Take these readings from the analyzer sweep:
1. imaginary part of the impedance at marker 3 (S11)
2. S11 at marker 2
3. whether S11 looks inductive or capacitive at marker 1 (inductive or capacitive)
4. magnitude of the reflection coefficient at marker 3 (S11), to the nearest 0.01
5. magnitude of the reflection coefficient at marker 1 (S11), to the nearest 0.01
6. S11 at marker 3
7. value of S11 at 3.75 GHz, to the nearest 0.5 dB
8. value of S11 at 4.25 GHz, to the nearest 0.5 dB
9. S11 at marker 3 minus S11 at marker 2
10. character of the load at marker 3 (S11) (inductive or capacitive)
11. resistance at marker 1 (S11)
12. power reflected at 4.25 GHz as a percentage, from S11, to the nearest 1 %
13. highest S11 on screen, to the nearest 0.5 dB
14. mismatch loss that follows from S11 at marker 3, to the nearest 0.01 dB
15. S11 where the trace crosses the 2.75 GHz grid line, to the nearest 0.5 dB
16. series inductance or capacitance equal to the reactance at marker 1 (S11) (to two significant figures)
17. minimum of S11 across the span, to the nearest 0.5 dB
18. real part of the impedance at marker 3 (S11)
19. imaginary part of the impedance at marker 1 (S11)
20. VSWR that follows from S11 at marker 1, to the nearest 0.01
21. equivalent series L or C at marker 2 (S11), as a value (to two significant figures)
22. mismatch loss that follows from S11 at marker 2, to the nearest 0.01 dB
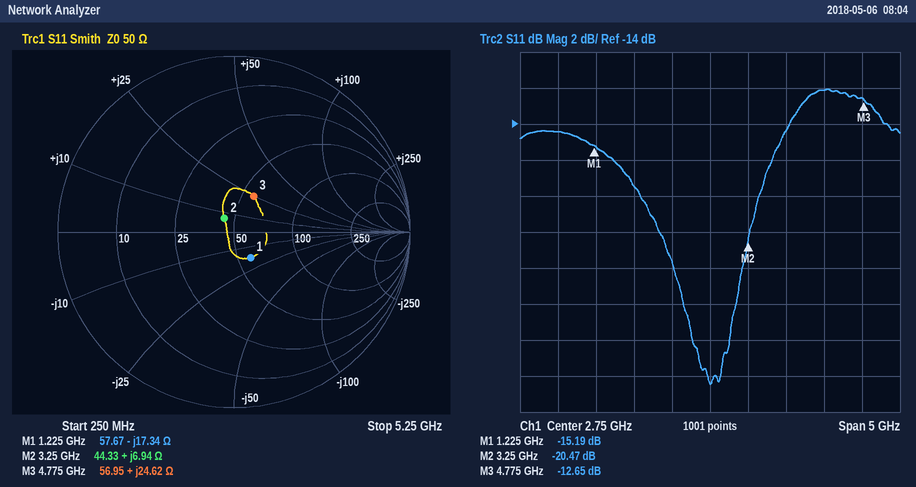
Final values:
+24.62 Ω
-20.47 dB
capacitive
0.23
0.17
-12.65 dB
-14.5 dB
-12.0 dB
7.82 dB
inductive
57.67 Ω
6 %
-12.0 dB
0.24 dB
-28.5 dB
7.5 pF
-28.5 dB
56.95 Ω
-17.34 Ω
1.42
340 pH
0.04 dB
